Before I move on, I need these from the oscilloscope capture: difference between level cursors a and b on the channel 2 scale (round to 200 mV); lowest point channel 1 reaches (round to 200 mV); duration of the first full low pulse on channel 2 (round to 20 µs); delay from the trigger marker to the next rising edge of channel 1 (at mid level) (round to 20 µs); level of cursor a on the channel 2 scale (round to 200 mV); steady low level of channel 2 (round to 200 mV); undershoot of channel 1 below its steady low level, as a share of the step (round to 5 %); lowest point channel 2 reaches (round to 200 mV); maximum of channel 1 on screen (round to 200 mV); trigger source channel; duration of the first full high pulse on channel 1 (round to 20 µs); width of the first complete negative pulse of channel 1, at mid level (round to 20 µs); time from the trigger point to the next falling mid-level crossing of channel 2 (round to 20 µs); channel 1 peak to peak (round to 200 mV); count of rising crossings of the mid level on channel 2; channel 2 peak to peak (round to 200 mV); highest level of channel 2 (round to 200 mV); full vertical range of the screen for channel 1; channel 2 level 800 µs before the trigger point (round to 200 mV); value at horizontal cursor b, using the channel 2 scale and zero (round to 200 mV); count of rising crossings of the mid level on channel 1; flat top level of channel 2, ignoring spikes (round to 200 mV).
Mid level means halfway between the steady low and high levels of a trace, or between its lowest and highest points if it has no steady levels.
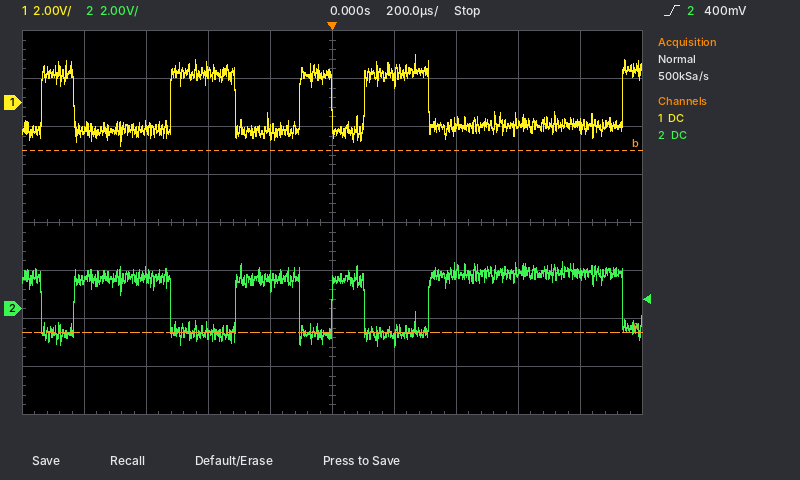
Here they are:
7.6 V
-1.8 V
100 µs
100 µs
-1.0 V
-1.0 V
30 %
-1.6 V
2.0 V
channel 2
100 µs
320 µs
100 µs
3.8 V
4
3.6 V
2.0 V
16 V
1.2 V
6.6 V
5
1.4 V
